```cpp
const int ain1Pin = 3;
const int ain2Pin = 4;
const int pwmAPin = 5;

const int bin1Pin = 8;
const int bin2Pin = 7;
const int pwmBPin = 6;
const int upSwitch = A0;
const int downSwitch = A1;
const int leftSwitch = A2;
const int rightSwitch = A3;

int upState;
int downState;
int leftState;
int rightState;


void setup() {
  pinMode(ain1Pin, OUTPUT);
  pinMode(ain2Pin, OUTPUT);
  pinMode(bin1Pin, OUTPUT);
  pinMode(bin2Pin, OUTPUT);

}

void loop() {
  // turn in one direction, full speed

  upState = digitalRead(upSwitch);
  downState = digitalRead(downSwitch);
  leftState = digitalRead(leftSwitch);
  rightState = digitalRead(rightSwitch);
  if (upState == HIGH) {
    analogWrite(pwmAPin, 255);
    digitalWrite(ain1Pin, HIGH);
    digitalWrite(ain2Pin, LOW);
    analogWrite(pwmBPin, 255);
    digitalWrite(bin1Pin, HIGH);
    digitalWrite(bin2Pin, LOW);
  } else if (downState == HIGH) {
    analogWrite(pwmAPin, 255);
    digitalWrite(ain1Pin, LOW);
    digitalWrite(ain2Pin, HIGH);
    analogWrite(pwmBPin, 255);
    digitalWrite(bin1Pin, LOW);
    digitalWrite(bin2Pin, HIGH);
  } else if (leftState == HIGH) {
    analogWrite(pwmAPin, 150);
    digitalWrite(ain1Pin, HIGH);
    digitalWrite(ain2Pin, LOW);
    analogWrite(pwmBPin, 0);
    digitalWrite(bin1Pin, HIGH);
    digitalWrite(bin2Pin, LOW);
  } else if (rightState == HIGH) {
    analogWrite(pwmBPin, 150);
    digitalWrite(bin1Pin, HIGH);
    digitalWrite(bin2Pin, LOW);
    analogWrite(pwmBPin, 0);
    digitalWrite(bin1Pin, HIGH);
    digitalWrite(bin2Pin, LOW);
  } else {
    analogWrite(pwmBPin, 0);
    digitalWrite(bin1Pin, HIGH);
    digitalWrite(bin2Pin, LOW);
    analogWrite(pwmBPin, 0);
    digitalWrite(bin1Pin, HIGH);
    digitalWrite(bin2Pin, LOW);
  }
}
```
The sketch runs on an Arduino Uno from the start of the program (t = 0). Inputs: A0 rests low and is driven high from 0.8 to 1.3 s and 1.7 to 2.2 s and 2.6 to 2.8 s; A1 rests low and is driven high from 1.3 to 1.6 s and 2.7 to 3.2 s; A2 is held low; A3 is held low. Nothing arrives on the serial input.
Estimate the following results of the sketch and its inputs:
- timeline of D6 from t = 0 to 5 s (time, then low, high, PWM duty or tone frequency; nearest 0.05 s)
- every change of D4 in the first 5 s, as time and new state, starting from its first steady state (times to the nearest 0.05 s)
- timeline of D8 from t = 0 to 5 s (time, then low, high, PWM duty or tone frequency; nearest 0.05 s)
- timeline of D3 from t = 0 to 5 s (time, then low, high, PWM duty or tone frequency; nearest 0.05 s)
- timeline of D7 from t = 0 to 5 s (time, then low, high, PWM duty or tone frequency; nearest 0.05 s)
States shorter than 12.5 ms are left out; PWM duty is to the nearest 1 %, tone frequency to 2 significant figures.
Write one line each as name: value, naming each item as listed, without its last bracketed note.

timeline of D6 from t = 0 to 5 s: 0 s low; 0.8 s high; 1.6 s low; 1.7 s high; 2.2 s low; 2.6 s high; 3.2 s low
every change of D4 in the first 5 s, as time and new state, starting from its first steady state: 0 s low; 1.3 s high; 1.7 s low; 2.8 s high
timeline of D8 from t = 0 to 5 s: 0 s high; 1.3 s low; 1.6 s high; 2.8 s low; 3.2 s high
timeline of D3 from t = 0 to 5 s: 0 s low; 0.8 s high; 1.3 s low; 1.7 s high; 2.8 s low
timeline of D7 from t = 0 to 5 s: 0 s low; 1.3 s high; 1.6 s low; 2.8 s high; 3.2 s low
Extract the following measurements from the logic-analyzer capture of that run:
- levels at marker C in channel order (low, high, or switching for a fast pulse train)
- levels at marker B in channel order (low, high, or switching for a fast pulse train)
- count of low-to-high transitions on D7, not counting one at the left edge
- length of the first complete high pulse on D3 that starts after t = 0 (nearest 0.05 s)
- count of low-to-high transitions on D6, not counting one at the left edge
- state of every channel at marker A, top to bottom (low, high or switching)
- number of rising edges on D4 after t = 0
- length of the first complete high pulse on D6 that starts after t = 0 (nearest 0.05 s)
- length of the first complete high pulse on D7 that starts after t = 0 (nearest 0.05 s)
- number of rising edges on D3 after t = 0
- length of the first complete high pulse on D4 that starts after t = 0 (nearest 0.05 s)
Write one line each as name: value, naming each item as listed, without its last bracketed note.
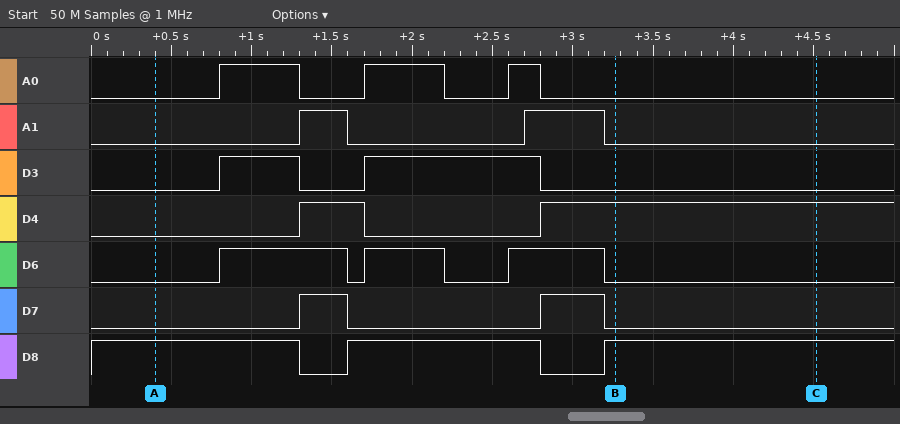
levels at marker C in channel order: A0 low, A1 low, D3 low, D4 high, D6 low, D7 low, D8 high
levels at marker B in channel order: A0 low, A1 low, D3 low, D4 high, D6 low, D7 low, D8 high
count of low-to-high transitions on D7, not counting one at the left edge: 2
length of the first complete high pulse on D3 that starts after t = 0: 0.50 s
count of low-to-high transitions on D6, not counting one at the left edge: 3
state of every channel at marker A, top to bottom: A0 low, A1 low, D3 low, D4 low, D6 low, D7 low, D8 high
number of rising edges on D4 after t = 0: 2
length of the first complete high pulse on D6 that starts after t = 0: 0.80 s
length of the first complete high pulse on D7 that starts after t = 0: 0.30 s
number of rising edges on D3 after t = 0: 2
length of the first complete high pulse on D4 that starts after t = 0: 0.40 s
